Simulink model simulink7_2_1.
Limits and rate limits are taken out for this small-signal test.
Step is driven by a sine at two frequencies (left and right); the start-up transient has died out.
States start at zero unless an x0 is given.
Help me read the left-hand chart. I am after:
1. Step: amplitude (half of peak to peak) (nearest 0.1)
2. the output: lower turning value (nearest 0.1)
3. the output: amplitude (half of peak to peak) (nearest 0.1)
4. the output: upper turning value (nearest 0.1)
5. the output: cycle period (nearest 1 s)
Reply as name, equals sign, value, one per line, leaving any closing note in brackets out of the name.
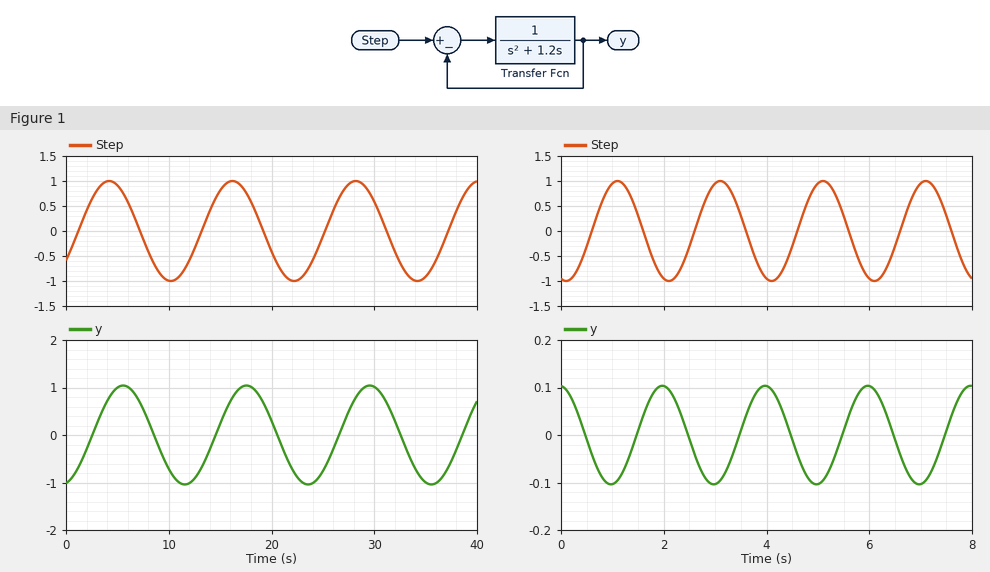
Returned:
Step: amplitude (half of peak to peak) = 1.0
the output: lower turning value = -1.0
the output: amplitude (half of peak to peak) = 1.0
the output: upper turning value = 1.0
the output: cycle period = 12 s
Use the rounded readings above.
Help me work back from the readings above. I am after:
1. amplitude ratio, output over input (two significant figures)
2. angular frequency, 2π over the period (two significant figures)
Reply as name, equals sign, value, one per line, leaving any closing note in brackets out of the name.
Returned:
amplitude ratio, output over input = 1.0
angular frequency, 2π over the period = 0.52 rad/s
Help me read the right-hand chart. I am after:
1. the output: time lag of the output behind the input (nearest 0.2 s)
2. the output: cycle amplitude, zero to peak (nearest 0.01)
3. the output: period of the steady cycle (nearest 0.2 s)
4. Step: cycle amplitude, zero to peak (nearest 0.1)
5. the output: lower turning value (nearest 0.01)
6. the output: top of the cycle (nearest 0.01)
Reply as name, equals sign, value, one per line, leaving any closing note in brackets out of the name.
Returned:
the output: time lag of the output behind the input = 0.8 s
the output: cycle amplitude, zero to peak = 0.10
the output: period of the steady cycle = 2.0 s
Step: cycle amplitude, zero to peak = 1.0
the output: lower turning value = -0.10
the output: top of the cycle = 0.10
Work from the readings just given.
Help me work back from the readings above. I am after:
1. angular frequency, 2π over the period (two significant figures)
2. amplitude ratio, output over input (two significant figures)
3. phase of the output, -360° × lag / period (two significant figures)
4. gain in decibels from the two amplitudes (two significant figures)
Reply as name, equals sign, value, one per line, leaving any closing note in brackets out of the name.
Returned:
angular frequency, 2π over the period = 3.1 rad/s
amplitude ratio, output over input = 0.10
phase of the output, -360° × lag / period = -140°
gain in decibels from the two amplitudes = -20 dB
